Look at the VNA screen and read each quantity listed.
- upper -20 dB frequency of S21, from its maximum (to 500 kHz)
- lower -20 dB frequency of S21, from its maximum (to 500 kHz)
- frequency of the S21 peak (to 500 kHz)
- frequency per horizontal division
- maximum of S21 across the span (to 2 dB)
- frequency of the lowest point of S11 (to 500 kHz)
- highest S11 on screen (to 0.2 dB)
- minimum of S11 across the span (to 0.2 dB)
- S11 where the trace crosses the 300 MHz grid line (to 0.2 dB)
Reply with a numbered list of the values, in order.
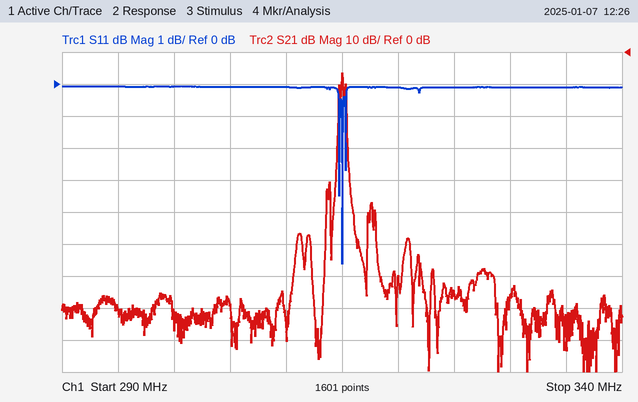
1. 315.5 MHz
2. 314.5 MHz
3. 315.0 MHz
4. 5 MHz
5. -6 dB
6. 315.0 MHz
7. 0.0 dB
8. -5.6 dB
9. 0.0 dB
